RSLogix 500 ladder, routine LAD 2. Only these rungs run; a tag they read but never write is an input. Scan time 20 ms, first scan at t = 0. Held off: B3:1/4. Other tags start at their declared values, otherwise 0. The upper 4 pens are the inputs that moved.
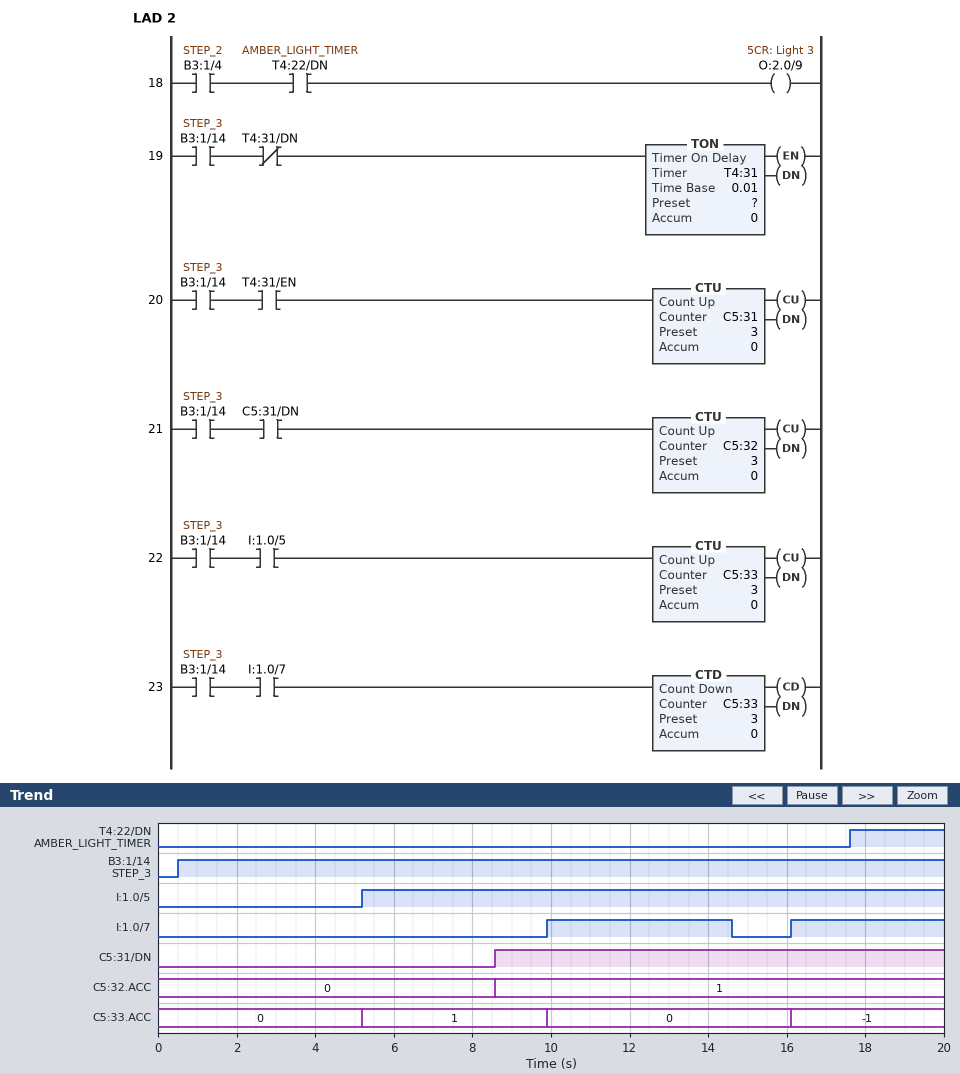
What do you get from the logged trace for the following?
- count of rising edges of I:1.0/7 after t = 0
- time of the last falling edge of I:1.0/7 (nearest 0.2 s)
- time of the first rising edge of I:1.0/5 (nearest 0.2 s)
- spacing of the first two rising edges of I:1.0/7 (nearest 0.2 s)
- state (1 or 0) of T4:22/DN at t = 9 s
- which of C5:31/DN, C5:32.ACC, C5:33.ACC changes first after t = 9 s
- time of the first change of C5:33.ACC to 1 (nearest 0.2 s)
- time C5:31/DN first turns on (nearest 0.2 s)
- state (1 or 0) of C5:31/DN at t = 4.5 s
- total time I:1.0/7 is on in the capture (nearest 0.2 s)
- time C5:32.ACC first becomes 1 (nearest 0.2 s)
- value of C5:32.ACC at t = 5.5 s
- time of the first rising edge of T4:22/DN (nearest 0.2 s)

2
14.6 s
5.2 s
6.2 s
0
C5:33.ACC
5.2 s
8.6 s
0
8.6 s
8.6 s
0
17.6 s
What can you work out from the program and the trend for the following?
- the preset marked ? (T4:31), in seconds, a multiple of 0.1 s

4.0 s
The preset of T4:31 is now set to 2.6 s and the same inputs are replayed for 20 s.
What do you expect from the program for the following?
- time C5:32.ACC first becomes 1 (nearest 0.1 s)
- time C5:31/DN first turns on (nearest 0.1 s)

5.8 s
5.8 s
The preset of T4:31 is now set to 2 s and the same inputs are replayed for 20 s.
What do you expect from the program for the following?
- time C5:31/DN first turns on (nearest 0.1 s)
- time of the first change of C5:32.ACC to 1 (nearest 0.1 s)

4.6 s
4.6 s
